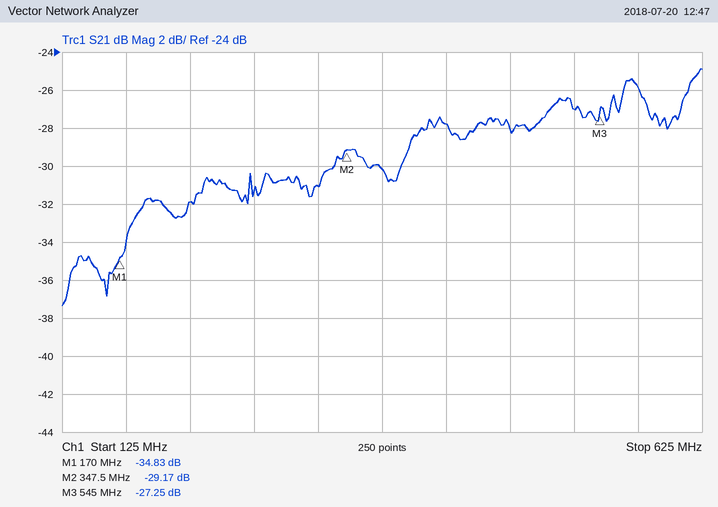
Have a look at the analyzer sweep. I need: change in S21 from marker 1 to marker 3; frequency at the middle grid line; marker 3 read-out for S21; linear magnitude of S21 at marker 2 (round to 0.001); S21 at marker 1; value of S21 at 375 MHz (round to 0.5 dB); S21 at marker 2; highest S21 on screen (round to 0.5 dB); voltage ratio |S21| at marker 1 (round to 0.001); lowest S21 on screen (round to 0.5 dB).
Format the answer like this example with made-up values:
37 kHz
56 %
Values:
7.58 dB
375 MHz
-27.25 dB
0.035
-34.83 dB
-30.0 dB
-29.17 dB
-25.0 dB
0.018
-37.5 dB
